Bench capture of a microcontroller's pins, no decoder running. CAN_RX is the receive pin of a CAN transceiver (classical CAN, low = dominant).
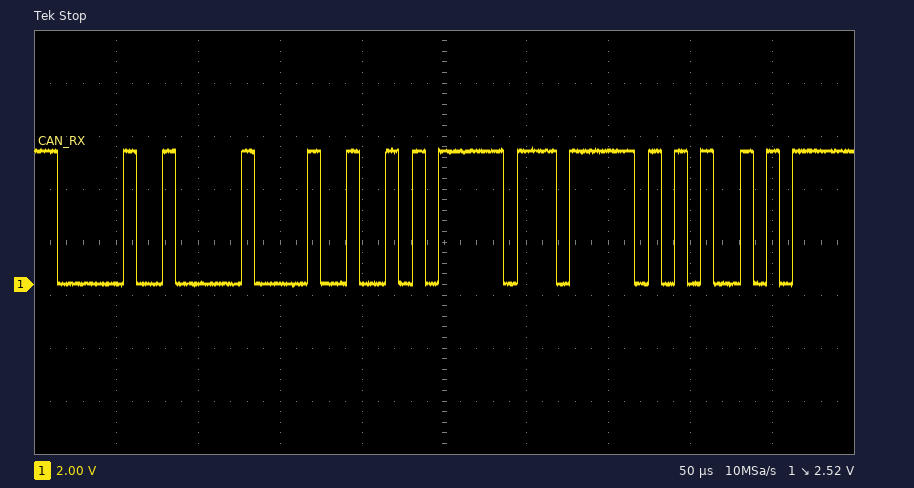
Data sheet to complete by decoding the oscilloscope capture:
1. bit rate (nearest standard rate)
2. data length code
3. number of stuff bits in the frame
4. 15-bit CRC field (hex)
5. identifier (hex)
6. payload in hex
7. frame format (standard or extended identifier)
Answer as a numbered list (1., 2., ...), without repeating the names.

1. 125 kbit/s
2. 2
3. 4
4. 0x3F52
5. 0x010
6. 4A FF
7. standard
